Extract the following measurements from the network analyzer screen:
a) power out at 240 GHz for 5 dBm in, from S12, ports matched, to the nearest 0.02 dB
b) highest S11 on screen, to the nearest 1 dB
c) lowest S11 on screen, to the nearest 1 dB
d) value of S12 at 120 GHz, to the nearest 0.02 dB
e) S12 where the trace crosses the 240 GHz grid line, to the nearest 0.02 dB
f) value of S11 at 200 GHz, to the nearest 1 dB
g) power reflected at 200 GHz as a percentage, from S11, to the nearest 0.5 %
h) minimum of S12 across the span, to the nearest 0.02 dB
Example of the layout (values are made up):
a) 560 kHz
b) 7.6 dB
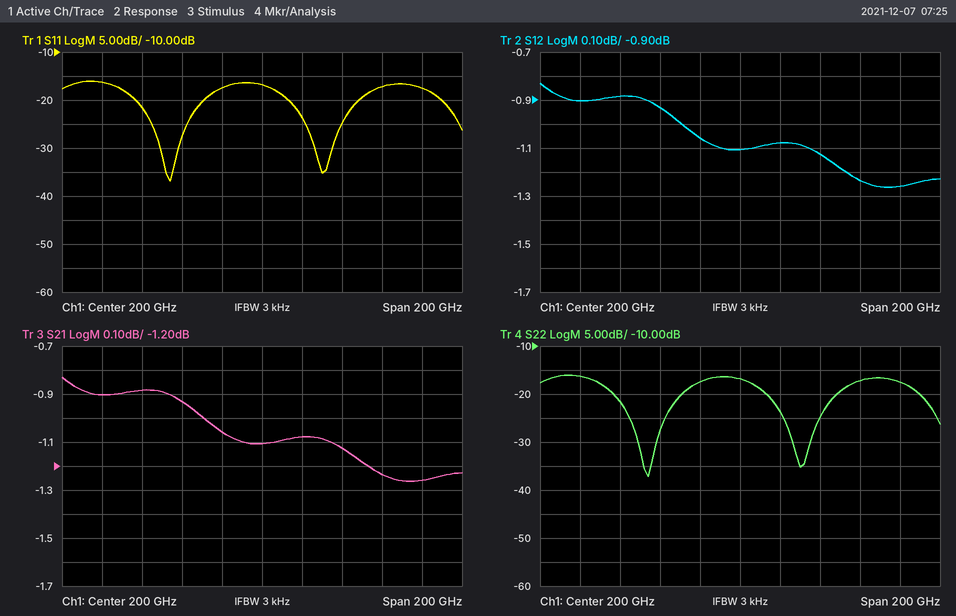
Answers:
a) 3.88 dBm
b) -16 dB
c) -37 dB
d) -0.90 dB
e) -1.12 dB
f) -17 dB
g) 2.0 %
h) -1.26 dB
